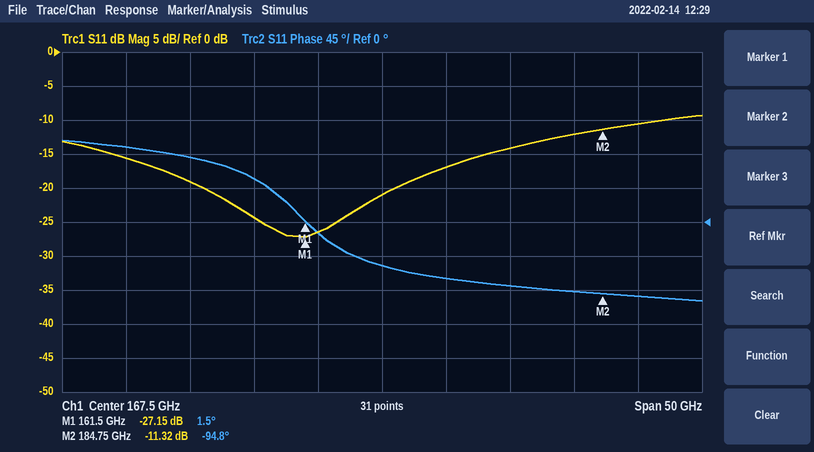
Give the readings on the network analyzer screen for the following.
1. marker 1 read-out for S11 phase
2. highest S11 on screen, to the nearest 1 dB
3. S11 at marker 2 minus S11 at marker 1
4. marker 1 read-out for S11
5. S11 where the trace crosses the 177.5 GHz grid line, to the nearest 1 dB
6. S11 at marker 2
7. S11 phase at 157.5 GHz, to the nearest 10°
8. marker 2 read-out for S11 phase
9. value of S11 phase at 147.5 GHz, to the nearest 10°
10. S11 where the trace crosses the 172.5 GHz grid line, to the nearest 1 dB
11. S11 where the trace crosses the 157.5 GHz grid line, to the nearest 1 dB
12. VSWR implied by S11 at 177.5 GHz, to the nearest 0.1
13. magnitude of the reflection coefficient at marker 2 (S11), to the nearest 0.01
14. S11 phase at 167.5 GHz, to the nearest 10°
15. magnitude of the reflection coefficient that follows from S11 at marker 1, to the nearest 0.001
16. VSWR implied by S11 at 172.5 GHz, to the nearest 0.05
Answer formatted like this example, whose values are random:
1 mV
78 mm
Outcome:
1.5°
-9 dB
15.83 dB
-27.15 dB
-14 dB
-11.32 dB
60°
-94.8°
100°
-17 dB
-24 dB
1.5
0.27
-60°
0.044
1.35
